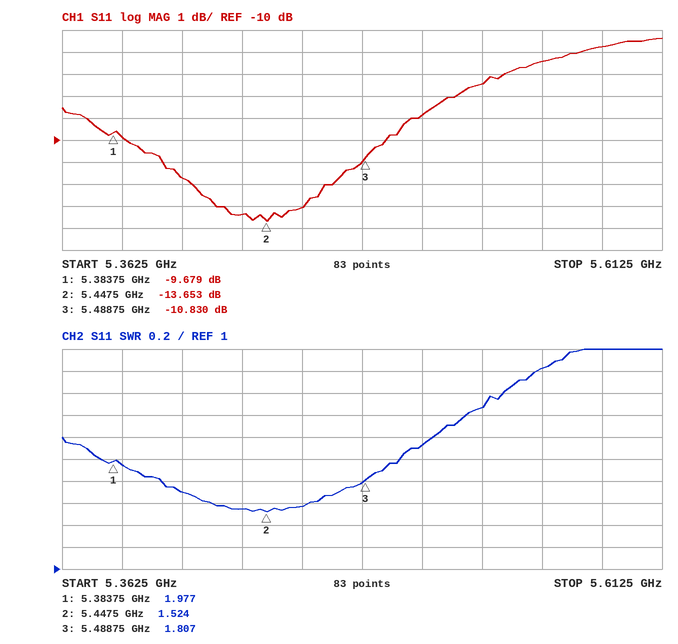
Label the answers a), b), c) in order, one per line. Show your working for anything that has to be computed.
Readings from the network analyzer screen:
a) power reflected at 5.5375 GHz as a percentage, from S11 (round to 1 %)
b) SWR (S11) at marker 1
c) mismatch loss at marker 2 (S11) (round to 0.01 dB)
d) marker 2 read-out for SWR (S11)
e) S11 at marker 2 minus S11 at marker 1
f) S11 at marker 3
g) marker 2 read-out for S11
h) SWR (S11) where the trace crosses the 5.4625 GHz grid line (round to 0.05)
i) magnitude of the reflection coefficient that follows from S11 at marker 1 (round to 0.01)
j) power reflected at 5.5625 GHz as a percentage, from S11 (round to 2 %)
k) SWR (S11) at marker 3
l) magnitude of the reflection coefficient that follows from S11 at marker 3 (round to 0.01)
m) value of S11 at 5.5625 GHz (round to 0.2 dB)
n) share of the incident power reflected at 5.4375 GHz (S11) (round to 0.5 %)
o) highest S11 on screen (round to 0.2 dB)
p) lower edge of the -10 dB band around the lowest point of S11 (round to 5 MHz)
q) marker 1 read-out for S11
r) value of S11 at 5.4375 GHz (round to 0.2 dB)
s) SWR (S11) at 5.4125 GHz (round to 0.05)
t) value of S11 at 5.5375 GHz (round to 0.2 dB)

a) 10^(-7.4/10) ≈ 18 %
b) 1.977
c) −10 log10(1 − 10^(-13.653/10)) ≈ 0.19 dB
d) 1.524
e) -13.653 − (-9.679) = -3.974 dB
f) -10.830 dB
g) -13.653 dB
h) 1.55
i) 10^(-9.679/20) ≈ 0.33
j) 10^(-6.4/10) ≈ 22.9 %, so 22 % to the nearest 2 %
k) 1.807
l) 10^(-10.83/20) ≈ 0.29
m) -6.4 dB
n) 10^(-13.4/10) ≈ 4.57 %, so 4.5 % to the nearest 0.5 %
o) -5.4 dB
p) 5.390 GHz
q) -9.679 dB
r) -13.4 dB
s) 1.70
t) -7.4 dB
